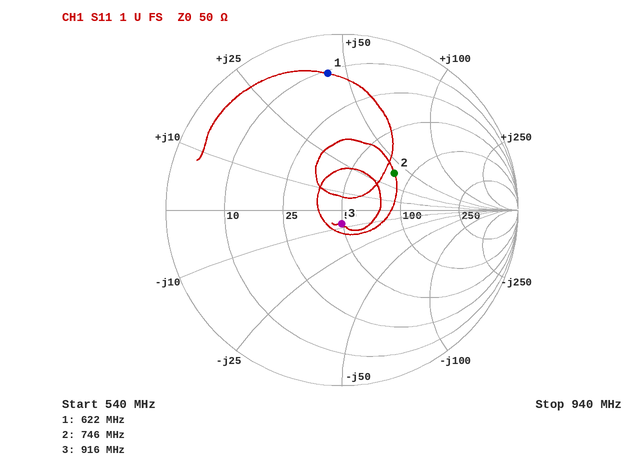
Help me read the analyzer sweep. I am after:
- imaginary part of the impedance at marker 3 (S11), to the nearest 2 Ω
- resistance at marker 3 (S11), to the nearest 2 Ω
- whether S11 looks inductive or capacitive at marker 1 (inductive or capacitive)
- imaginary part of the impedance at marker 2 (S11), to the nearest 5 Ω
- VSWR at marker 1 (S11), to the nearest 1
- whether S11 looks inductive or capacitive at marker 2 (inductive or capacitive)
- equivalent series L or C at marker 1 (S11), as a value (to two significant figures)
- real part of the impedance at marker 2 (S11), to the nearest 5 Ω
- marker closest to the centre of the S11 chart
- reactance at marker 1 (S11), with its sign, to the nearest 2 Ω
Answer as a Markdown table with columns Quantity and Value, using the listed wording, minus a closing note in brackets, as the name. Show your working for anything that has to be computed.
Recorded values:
| Quantity | Value |
|---|---|
| imaginary part of the impedance at marker 3 (S11), to the nearest 2 Ω | -8 Ω |
| resistance at marker 3 (S11), to the nearest 2 Ω | 50 Ω |
| whether S11 looks inductive or capacitive at marker 1 | inductive |
| imaginary part of the impedance at marker 2 (S11), to the nearest 5 Ω | +40 Ω |
| VSWR at marker 1 (S11), to the nearest 1 | 8 |
| whether S11 looks inductive or capacitive at marker 2 | inductive |
| equivalent series L or C at marker 1 (S11), as a value | L = 44 Ω/(2π × 622 MHz) ≈ 11 nH |
| real part of the impedance at marker 2 (S11), to the nearest 5 Ω | 80 Ω |
| marker closest to the centre of the S11 chart | marker 3 |
| reactance at marker 1 (S11), with its sign, to the nearest 2 Ω | +44 Ω |
